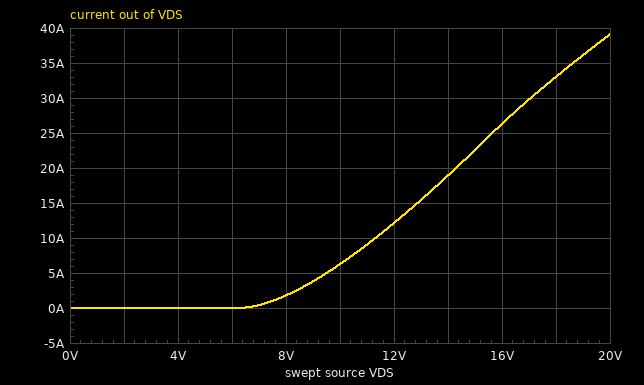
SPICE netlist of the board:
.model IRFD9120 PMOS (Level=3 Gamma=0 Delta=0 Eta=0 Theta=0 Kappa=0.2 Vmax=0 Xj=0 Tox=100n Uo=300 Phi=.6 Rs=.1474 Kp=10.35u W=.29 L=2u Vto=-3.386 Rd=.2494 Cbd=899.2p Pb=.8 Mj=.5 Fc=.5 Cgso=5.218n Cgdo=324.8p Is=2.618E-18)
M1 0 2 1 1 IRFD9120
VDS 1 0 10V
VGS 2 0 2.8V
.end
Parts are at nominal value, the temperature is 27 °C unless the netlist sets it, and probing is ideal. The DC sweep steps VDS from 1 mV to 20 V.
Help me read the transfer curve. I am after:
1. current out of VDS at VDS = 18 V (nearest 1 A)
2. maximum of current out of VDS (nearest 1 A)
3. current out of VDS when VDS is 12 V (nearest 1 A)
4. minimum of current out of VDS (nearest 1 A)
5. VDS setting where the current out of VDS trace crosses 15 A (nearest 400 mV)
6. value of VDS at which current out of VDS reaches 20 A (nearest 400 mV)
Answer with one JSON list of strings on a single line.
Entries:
["33 A", "39 A", "12 A", "0 A", "12.8 V", "14.4 V"]
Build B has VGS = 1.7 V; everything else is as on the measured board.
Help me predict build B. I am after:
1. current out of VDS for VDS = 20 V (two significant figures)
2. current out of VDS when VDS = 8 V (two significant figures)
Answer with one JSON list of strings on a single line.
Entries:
["41 A", "4.0 A"]
